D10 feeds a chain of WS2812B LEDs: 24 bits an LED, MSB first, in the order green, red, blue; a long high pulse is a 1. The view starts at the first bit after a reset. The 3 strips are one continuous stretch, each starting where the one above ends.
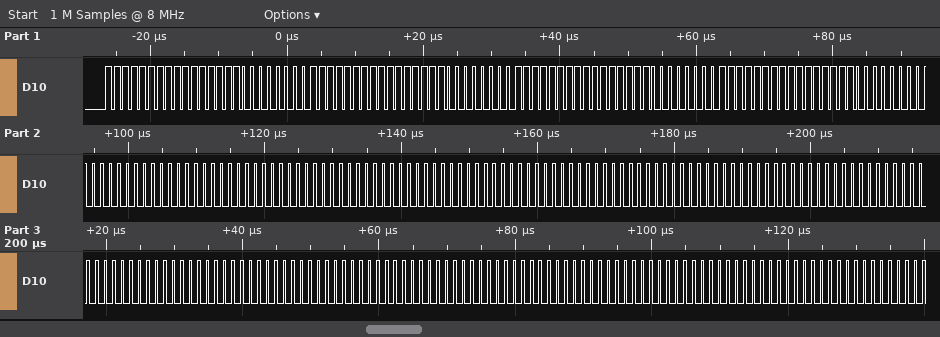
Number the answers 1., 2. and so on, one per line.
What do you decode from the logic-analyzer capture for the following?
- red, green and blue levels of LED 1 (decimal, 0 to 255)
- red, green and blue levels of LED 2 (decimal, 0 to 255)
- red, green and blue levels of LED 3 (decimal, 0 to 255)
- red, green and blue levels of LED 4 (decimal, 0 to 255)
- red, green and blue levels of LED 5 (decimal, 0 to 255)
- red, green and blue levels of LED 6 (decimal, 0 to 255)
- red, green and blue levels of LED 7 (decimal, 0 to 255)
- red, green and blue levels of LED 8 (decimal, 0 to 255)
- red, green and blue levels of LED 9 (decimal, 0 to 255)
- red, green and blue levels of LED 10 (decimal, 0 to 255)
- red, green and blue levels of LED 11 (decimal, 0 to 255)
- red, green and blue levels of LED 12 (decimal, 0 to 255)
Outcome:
1. 255, 255, 0
2. 255, 255, 0
3. 255, 255, 0
4. 255, 255, 0
5. 0, 0, 0
6. 0, 0, 0
7. 0, 0, 0
8. 0, 0, 0
9. 0, 0, 0
10. 0, 0, 0
11. 0, 0, 0
12. 0, 0, 0
